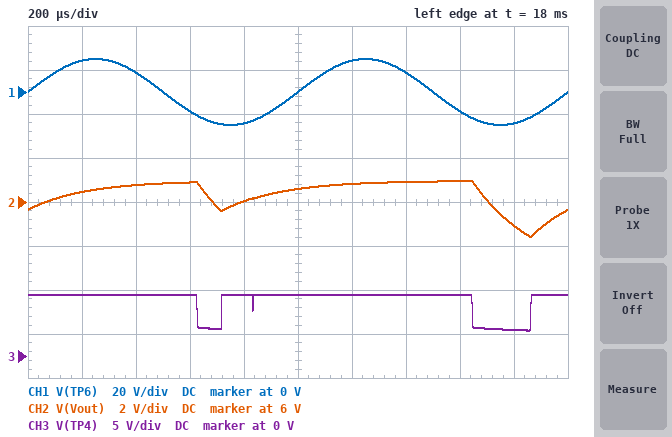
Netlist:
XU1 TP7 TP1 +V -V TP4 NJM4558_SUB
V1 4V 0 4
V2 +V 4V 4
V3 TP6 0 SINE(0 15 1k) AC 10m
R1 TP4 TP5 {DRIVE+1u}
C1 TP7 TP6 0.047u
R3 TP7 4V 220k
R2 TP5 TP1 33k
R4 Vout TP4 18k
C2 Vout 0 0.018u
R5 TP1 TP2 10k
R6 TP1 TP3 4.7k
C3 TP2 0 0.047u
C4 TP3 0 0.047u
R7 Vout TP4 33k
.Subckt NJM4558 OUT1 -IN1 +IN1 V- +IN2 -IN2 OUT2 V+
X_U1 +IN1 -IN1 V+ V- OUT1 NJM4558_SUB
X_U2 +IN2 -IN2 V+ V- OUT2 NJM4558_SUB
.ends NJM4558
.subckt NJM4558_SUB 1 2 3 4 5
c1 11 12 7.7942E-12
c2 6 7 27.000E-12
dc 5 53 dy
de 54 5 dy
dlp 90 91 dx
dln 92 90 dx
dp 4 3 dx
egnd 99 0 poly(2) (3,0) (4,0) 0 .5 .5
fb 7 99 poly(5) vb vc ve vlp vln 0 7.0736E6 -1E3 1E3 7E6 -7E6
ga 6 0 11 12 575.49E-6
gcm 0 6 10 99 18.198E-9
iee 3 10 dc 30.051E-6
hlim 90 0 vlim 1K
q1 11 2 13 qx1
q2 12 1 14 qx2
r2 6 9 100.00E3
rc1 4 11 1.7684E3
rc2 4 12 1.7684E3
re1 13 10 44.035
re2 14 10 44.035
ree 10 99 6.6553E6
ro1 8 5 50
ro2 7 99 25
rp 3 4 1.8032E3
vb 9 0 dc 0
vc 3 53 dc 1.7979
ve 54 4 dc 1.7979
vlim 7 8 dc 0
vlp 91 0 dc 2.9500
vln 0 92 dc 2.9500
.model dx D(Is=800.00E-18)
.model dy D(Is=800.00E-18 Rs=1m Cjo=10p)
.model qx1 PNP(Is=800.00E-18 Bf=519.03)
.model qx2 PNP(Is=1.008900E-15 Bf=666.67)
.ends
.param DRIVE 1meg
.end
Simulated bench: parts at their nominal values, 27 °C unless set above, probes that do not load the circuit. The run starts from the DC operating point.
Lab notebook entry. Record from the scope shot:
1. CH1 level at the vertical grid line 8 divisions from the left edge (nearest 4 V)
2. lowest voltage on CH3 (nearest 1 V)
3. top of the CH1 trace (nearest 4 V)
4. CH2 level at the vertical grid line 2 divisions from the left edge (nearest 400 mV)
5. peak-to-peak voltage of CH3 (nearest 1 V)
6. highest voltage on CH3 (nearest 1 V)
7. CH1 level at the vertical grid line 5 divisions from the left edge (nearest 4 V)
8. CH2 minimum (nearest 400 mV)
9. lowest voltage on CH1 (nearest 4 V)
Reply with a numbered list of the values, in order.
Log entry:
1. -8 V
2. 3 V
3. 16 V
4. 6.8 V
5. 4 V
6. 7 V
7. 0 V
8. 4.4 V
9. -16 V
